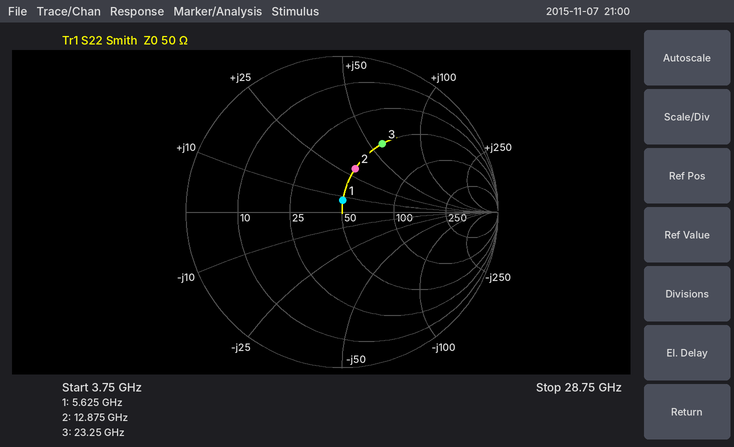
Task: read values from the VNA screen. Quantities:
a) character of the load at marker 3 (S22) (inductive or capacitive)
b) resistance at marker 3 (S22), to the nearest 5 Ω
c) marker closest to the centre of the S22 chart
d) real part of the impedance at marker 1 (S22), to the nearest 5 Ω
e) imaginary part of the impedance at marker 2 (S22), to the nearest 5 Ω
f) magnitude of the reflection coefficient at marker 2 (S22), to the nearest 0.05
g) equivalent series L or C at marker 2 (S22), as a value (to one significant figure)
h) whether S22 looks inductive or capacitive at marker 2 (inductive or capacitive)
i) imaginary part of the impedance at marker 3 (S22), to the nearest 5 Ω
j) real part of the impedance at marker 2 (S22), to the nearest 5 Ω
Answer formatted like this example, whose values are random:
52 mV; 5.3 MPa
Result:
inductive; 50 Ω; marker 1; 50 Ω; +30 Ω; 0.30; 400 pH; inductive; +60 Ω; 50 Ω
